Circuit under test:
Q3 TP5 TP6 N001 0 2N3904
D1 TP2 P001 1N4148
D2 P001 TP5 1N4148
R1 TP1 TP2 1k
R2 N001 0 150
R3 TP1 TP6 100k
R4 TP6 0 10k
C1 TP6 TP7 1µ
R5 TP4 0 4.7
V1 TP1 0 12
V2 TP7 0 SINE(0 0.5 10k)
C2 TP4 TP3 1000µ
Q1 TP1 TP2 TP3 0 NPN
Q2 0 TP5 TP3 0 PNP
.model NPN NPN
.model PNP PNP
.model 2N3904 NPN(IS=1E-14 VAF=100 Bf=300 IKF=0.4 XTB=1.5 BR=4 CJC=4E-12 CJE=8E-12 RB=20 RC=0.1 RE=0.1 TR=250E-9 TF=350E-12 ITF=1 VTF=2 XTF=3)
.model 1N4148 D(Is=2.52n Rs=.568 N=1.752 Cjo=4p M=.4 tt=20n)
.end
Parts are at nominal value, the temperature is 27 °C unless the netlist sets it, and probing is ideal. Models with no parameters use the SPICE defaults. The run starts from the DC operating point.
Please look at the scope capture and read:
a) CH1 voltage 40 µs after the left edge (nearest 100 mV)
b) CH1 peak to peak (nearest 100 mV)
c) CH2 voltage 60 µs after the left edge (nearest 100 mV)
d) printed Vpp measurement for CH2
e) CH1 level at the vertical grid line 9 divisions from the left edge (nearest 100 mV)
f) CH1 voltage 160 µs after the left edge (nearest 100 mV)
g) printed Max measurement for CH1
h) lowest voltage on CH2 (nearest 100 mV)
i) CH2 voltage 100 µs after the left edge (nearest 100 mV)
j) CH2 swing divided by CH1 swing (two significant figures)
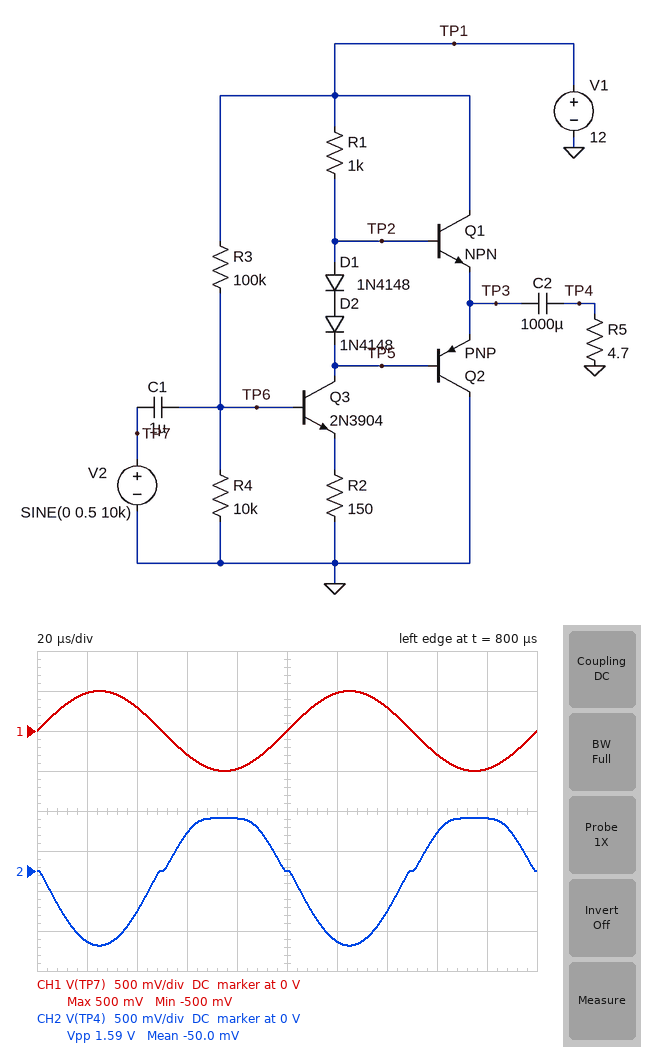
300 mV
1.0 V
500 mV
1.59 V
-500 mV
-300 mV
500 mV
-900 mV
0 V
1.6
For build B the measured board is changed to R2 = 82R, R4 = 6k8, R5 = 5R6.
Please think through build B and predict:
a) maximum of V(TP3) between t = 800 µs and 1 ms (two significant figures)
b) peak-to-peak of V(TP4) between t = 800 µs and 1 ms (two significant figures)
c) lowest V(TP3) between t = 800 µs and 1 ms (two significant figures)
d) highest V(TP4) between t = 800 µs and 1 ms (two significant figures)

11 V
2.2 V
8.4 V
310 mV
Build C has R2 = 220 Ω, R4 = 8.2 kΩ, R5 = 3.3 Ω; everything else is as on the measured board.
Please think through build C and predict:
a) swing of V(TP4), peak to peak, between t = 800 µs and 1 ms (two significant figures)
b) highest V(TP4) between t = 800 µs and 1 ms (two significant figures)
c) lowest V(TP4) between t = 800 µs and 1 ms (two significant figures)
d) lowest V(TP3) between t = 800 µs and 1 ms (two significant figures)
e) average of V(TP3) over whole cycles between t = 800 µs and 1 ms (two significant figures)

650 mV
190 mV
-460 mV
9.9 V
10 V
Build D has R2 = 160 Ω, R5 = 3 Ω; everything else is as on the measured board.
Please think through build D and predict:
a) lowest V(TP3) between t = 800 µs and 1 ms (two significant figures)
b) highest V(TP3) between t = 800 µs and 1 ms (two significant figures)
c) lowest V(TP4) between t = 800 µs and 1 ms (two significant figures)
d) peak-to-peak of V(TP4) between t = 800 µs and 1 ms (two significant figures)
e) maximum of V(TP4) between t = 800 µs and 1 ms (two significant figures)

8.5 V
9.6 V
-630 mV
1.1 V
450 mV
